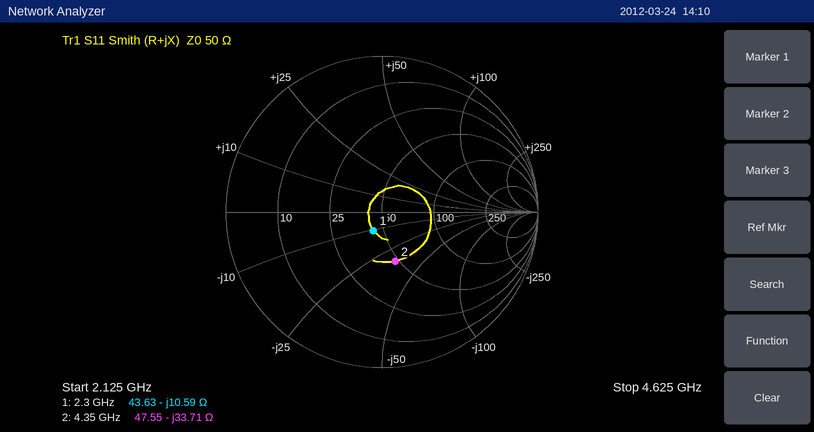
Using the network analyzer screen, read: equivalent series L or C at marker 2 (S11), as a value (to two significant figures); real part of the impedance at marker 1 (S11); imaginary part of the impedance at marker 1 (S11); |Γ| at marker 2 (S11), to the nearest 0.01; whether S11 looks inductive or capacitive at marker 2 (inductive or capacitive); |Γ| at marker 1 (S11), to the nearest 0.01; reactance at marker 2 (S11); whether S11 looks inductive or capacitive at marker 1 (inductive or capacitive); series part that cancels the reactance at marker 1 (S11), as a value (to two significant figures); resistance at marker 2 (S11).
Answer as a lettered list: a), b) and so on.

a) 1.1 pF
b) 43.63 Ω
c) -10.59 Ω
d) 0.33
e) capacitive
f) 0.13
g) -33.71 Ω
h) capacitive
i) 730 pH
j) 47.55 Ω
